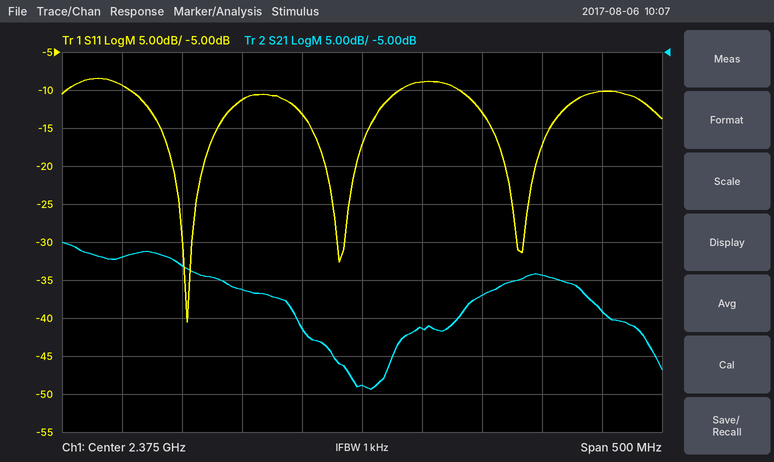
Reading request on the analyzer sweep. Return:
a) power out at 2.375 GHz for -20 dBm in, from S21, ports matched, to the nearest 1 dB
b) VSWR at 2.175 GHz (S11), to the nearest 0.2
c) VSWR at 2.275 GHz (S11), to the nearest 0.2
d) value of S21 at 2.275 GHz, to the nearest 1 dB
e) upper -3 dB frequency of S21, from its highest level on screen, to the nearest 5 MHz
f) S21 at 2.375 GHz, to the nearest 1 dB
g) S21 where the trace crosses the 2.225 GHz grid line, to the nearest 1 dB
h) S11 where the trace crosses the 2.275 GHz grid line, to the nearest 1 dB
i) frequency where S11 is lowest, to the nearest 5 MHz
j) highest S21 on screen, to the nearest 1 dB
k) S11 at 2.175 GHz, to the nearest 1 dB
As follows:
-69 dBm
2.0
1.8
-36 dB
2.225 GHz
-49 dB
-33 dB
-11 dB
2.230 GHz
-30 dB
-9 dB
